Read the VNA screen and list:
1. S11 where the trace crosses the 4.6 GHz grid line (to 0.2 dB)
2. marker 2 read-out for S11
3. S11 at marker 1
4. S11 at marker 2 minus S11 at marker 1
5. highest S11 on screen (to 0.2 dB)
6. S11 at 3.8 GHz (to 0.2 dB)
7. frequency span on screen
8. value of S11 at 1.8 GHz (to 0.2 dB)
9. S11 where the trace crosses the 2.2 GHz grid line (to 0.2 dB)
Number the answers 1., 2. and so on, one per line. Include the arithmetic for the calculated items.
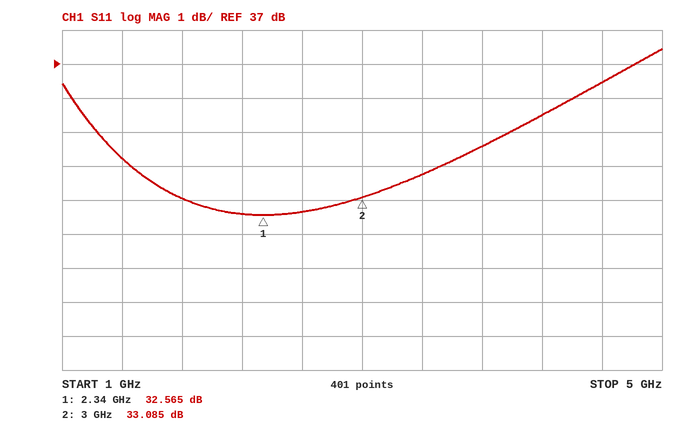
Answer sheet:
1. 36.4 dB
2. 33.085 dB
3. 32.565 dB
4. 33.085 − (32.565) = 0.520 dB
5. 37.4 dB
6. 34.6 dB
7. 4 GHz
8. 33.0 dB
9. 32.6 dB
